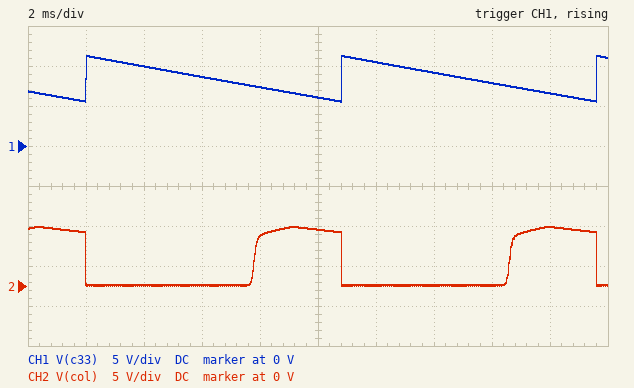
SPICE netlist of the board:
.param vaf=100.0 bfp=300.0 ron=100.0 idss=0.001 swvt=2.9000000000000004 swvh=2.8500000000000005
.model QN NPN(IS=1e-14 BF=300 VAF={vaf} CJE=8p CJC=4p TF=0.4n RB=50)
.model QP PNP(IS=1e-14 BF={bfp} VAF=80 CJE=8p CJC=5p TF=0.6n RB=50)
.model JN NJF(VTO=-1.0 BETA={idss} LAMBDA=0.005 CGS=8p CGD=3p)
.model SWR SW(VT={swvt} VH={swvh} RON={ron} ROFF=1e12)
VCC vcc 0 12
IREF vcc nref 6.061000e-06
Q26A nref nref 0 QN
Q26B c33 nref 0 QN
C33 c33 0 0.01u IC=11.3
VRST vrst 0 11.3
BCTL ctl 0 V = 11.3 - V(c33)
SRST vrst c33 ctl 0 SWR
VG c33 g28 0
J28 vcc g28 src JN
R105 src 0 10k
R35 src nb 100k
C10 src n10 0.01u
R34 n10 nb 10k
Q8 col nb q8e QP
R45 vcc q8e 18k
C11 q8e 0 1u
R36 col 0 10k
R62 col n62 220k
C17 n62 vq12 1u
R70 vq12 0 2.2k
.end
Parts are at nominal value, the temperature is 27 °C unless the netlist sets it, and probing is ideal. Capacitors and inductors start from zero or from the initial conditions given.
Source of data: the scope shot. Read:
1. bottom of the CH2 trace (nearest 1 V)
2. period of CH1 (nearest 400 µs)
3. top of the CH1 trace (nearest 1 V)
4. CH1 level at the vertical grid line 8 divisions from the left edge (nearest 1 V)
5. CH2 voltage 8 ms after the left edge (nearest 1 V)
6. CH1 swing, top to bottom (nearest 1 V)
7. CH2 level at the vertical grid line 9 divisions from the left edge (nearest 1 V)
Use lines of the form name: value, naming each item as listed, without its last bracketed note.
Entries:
bottom of the CH2 trace: 0 V
period of CH1: 8.8 ms
top of the CH1 trace: 11 V
CH1 level at the vertical grid line 8 divisions from the left edge: 8 V
CH2 voltage 8 ms after the left edge: 6 V
CH1 swing, top to bottom: 6 V
CH2 level at the vertical grid line 9 divisions from the left edge: 7 V
